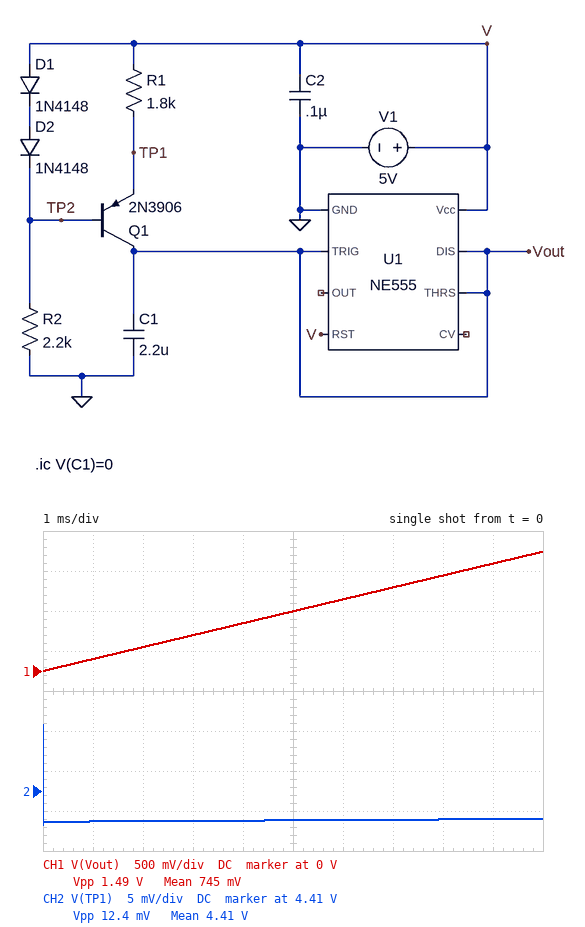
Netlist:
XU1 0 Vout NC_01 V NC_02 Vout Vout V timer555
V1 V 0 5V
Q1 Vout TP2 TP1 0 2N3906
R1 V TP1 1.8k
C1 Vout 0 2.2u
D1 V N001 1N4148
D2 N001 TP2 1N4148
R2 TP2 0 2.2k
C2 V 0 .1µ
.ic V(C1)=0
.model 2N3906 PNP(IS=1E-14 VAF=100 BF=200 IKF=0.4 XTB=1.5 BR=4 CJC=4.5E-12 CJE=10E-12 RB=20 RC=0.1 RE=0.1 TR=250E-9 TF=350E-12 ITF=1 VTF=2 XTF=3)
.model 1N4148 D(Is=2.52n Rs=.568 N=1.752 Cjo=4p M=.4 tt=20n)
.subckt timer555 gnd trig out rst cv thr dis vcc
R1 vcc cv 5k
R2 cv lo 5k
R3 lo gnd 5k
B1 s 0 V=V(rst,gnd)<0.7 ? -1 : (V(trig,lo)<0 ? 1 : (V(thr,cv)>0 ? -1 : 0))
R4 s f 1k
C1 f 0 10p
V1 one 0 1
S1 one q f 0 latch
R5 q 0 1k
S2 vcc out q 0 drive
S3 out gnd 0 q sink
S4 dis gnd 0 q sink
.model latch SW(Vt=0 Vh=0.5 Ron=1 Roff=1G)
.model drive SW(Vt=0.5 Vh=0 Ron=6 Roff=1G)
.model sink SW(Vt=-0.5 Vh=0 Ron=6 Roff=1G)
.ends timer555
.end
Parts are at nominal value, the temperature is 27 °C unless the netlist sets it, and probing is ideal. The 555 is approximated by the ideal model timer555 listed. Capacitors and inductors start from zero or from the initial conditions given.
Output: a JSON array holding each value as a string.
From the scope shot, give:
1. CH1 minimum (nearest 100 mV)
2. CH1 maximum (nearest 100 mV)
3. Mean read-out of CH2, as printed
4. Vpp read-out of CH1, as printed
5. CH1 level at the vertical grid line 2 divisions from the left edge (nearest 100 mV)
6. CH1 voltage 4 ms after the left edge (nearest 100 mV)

["0 V", "1.5 V", "4.41 V", "1.49 V", "300 mV", "600 mV"]
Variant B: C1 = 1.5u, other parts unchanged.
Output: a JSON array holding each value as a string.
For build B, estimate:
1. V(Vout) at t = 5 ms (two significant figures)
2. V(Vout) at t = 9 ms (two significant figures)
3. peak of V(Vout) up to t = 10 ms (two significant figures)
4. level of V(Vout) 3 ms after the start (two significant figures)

["1.1 V", "2.0 V", "2.2 V", "660 mV"]
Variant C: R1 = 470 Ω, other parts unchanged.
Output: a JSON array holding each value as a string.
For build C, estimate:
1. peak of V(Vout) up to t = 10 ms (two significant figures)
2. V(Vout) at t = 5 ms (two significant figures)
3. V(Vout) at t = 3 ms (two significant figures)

["3.3 V", "2.7 V", "1.6 V"]
